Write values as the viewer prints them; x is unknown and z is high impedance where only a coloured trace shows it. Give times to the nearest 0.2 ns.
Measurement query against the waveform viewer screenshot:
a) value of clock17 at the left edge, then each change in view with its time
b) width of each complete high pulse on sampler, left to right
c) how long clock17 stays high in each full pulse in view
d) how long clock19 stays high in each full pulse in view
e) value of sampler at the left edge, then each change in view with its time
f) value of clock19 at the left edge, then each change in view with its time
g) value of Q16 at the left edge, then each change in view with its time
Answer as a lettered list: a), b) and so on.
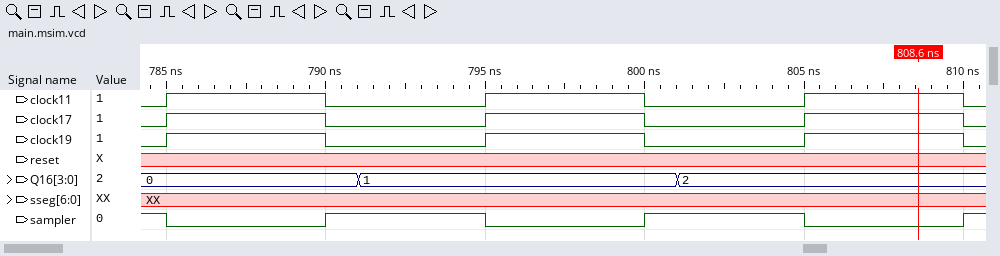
a) 0, 1 at 785 ns, 0 at 790 ns, 1 at 795 ns, 0 at 800 ns, 1 at 805 ns, 0 at 810 ns
b) 5 ns, 5 ns
c) 5 ns, 5 ns, 5 ns
d) 5 ns, 5 ns, 5 ns
e) 1, 0 at 785 ns, 1 at 790 ns, 0 at 795 ns, 1 at 800 ns, 0 at 805 ns, 1 at 810 ns
f) 0, 1 at 785 ns, 0 at 790 ns, 1 at 795 ns, 0 at 800 ns, 1 at 805 ns, 0 at 810 ns
g) 0, 1 at 791 ns, 2 at 801 ns
